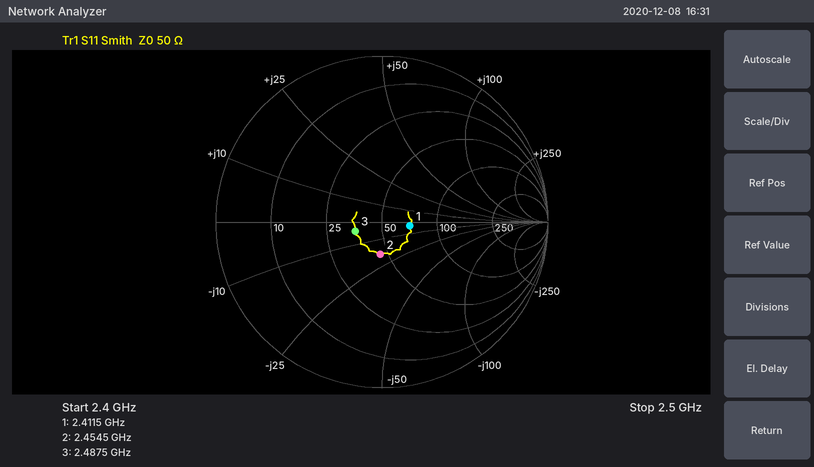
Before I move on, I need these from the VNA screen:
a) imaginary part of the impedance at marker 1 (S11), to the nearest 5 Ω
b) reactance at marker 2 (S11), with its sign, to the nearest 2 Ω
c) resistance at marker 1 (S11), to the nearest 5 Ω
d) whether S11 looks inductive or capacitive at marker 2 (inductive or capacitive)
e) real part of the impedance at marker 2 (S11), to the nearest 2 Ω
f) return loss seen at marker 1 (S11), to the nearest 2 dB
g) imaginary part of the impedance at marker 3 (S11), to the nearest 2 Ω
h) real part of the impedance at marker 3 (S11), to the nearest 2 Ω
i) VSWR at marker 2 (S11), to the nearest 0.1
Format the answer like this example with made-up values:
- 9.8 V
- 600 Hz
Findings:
- -5 Ω
- -18 Ω
- 70 Ω
- capacitive
- 46 Ω
- 16 dB
- -4 Ω
- 36 Ω
- 1.5
